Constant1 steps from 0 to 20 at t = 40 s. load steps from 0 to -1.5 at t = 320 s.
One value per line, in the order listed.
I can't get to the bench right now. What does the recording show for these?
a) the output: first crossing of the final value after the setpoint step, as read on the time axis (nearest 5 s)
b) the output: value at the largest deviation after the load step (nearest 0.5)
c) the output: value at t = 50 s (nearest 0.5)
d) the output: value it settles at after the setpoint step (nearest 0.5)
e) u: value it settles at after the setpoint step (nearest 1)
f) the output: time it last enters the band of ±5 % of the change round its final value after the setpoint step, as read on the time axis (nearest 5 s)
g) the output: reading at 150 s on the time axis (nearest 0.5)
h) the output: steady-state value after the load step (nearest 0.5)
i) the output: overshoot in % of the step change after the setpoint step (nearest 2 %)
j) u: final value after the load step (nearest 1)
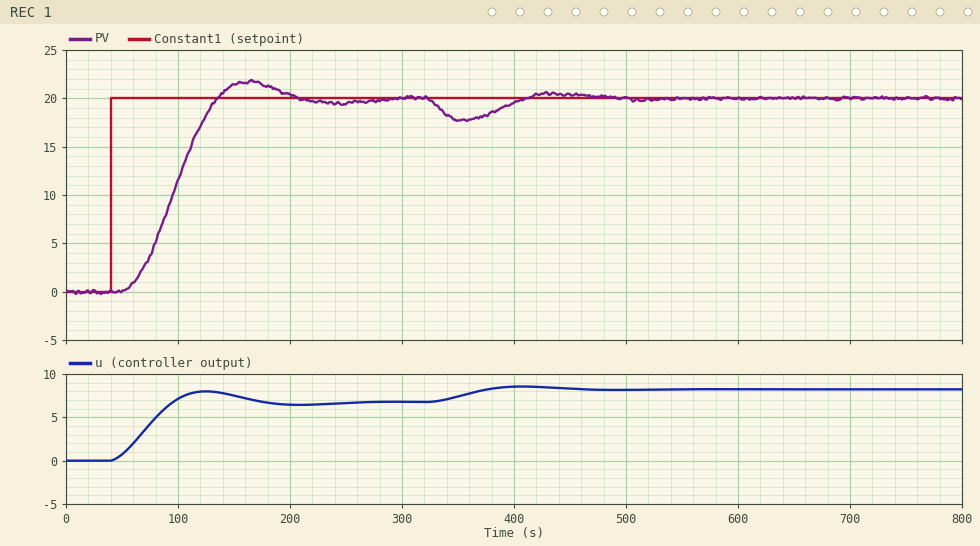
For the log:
135 s
17.5
0.0
20.0
7
185 s
21.5
20.0
8 %
8
